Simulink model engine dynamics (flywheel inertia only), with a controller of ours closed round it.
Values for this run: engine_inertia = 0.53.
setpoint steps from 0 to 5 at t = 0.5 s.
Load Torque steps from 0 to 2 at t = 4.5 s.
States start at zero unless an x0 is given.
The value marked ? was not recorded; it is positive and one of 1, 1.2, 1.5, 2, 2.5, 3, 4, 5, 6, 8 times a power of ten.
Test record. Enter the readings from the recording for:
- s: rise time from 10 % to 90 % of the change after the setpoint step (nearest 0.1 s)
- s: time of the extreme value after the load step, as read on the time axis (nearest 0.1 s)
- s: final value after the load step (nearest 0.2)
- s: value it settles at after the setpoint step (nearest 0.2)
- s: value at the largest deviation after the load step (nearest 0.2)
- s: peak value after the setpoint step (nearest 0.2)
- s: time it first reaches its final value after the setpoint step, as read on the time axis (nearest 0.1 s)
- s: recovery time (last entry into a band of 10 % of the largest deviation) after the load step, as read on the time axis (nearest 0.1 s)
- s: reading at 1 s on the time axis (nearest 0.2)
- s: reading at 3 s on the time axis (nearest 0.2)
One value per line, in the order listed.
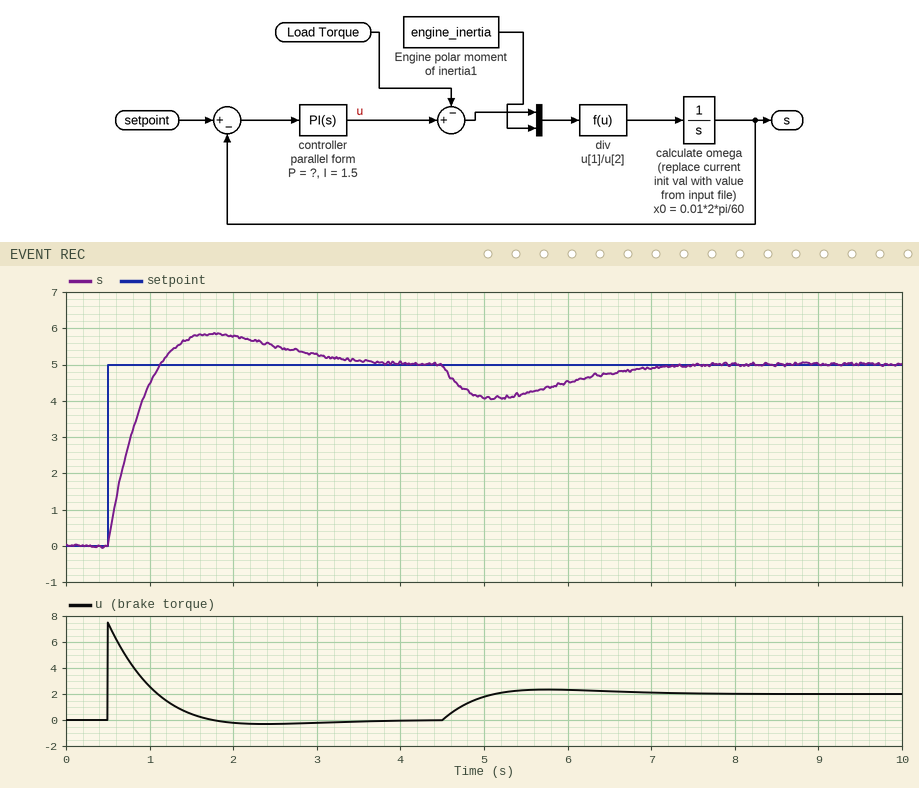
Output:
0.5 s
5.1 s
5.0
5.0
4.0
5.8
1.1 s
7.0 s
4.4
5.2
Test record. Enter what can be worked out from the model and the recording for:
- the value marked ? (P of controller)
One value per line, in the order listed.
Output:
1.5
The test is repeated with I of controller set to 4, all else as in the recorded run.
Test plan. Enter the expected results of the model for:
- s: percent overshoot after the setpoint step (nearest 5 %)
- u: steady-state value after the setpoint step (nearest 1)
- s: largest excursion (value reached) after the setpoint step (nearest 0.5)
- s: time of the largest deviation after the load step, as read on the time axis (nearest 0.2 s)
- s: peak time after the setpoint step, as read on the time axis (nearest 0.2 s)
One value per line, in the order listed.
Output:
30 %
0
6.5
5.0 s
1.4 s
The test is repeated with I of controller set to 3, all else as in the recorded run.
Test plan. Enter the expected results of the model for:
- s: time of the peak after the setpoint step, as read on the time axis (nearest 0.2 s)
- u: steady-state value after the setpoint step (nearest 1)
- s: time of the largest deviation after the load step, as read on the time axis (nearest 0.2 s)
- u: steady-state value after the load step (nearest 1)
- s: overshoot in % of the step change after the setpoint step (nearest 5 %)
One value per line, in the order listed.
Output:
1.4 s
0
5.0 s
2
25 %
